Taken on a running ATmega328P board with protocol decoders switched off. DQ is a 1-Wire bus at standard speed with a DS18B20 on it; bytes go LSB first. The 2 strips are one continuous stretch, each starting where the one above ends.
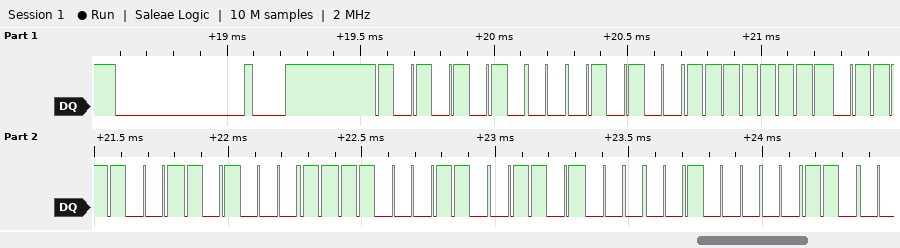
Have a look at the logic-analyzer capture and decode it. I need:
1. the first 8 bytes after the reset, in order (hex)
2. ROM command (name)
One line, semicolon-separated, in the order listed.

55 28 FF 9E C5 63 16 04; Match ROM
